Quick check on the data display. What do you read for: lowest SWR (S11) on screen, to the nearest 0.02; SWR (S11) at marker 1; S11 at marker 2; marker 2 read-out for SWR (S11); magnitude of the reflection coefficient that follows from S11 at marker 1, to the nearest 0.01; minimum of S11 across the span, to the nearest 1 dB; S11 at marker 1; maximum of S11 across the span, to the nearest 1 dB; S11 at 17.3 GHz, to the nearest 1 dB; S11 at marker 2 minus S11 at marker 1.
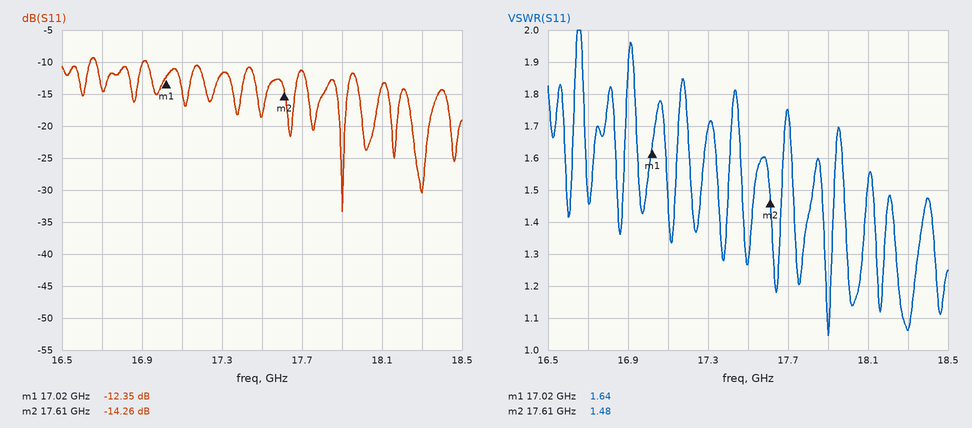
1.04
1.64
-14.26 dB
1.48
0.24
-33 dB
-12.35 dB
-9 dB
-12 dB
-1.91 dB
